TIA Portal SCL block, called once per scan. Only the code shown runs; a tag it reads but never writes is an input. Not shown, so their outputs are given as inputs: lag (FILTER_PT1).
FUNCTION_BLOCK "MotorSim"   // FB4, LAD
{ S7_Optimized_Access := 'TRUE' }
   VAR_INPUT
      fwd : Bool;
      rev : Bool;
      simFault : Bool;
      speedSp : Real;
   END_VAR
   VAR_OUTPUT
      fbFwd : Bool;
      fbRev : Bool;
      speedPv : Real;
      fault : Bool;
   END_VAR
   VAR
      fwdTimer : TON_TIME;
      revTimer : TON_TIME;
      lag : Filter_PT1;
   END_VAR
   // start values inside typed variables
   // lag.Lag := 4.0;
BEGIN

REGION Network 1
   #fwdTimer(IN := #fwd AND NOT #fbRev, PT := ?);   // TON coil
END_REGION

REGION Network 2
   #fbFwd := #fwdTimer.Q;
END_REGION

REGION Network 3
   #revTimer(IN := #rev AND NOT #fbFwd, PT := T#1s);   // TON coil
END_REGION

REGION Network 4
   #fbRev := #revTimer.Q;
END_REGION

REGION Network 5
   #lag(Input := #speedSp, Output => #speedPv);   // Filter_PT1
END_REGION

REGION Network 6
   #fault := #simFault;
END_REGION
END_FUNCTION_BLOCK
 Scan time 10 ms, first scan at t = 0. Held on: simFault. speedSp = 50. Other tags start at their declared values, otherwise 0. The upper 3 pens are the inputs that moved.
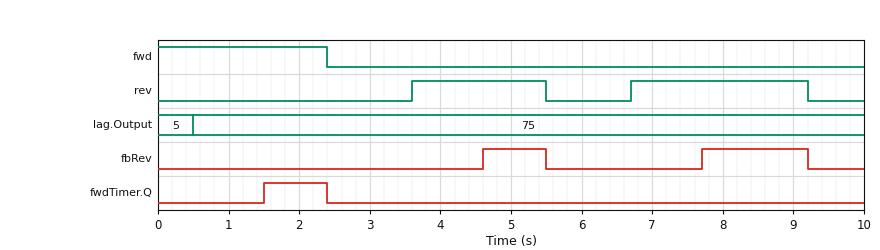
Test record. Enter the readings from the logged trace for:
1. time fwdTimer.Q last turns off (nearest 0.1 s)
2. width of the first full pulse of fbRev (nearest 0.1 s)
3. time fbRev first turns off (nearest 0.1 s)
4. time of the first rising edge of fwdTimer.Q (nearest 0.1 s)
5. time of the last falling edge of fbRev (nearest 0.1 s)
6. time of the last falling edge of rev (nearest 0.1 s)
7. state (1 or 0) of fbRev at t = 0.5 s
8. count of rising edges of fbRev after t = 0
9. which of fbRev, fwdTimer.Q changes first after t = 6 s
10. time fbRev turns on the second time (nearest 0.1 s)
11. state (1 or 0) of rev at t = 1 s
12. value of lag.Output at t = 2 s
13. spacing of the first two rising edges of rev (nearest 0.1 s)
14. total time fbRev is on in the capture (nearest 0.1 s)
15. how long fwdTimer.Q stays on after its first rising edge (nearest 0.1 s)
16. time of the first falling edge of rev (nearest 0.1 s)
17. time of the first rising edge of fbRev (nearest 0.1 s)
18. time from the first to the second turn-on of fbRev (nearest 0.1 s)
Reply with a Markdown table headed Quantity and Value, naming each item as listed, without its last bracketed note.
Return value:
| Quantity | Value |
|---|---|
| time fwdTimer.Q last turns off | 2.4 s |
| width of the first full pulse of fbRev | 0.9 s |
| time fbRev first turns off | 5.5 s |
| time of the first rising edge of fwdTimer.Q | 1.5 s |
| time of the last falling edge of fbRev | 9.2 s |
| time of the last falling edge of rev | 9.2 s |
| state (1 or 0) of fbRev at t = 0.5 s | 0 |
| count of rising edges of fbRev after t = 0 | 2 |
| which of fbRev, fwdTimer.Q changes first after t = 6 s | fbRev |
| time fbRev turns on the second time | 7.7 s |
| state (1 or 0) of rev at t = 1 s | 0 |
| value of lag.Output at t = 2 s | 75 |
| spacing of the first two rising edges of rev | 3.1 s |
| total time fbRev is on in the capture | 2.4 s |
| how long fwdTimer.Q stays on after its first rising edge | 0.9 s |
| time of the first falling edge of rev | 5.5 s |
| time of the first rising edge of fbRev | 4.6 s |
| time from the first to the second turn-on of fbRev | 3.1 s |
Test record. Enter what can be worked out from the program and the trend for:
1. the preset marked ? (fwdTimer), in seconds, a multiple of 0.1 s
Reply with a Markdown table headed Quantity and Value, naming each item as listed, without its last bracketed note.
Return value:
| Quantity | Value |
|---|---|
| the preset marked ? (fwdTimer), in seconds, a multiple of 0.1 s | 1.5 s |
